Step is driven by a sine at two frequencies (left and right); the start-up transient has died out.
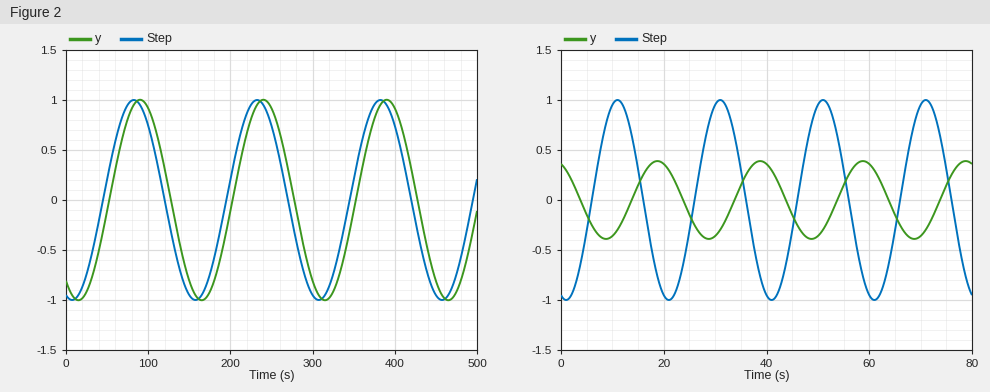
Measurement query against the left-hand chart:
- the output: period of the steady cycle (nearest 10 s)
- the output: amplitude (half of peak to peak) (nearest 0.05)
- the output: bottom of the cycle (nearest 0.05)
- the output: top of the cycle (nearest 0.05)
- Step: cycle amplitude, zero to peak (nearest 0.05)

150 s
1.00
-1.00
1.00
1.00
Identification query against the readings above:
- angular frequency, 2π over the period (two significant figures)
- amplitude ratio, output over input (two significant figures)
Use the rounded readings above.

0.042 rad/s
1.0
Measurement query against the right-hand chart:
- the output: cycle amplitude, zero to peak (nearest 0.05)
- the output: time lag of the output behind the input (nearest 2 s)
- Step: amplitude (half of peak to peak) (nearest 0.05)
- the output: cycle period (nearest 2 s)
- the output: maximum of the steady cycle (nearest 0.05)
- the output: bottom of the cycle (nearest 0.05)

0.40
8 s
1.00
20 s
0.40
-0.40
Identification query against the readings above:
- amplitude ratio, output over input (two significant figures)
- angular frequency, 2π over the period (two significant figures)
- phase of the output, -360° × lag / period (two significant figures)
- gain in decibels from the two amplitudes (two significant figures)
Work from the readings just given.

0.40
0.31 rad/s
-140°
-8.0 dB
